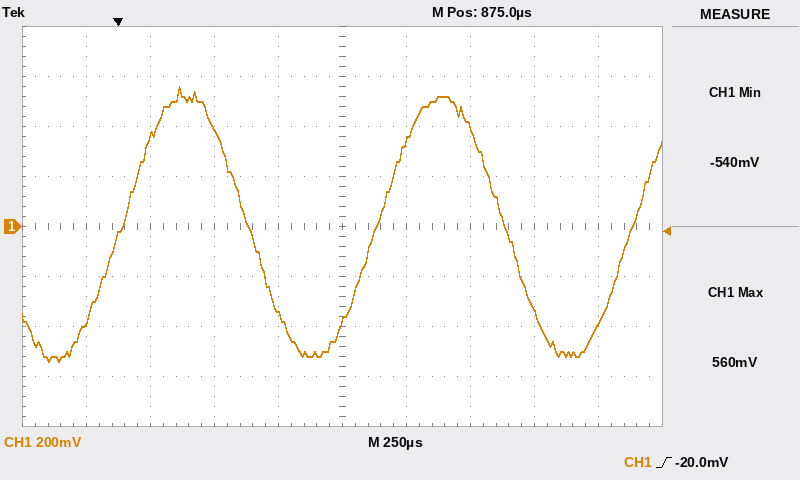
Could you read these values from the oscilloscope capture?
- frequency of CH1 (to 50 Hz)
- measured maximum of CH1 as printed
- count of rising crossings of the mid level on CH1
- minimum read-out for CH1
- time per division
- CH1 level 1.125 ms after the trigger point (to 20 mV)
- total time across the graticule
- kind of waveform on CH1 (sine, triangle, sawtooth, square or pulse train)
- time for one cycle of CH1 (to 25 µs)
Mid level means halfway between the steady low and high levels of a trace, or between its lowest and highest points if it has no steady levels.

1.00 kHz
560 mV
3
-540 mV
250 µs
340 mV
2.5 ms
sine
1.000 ms
